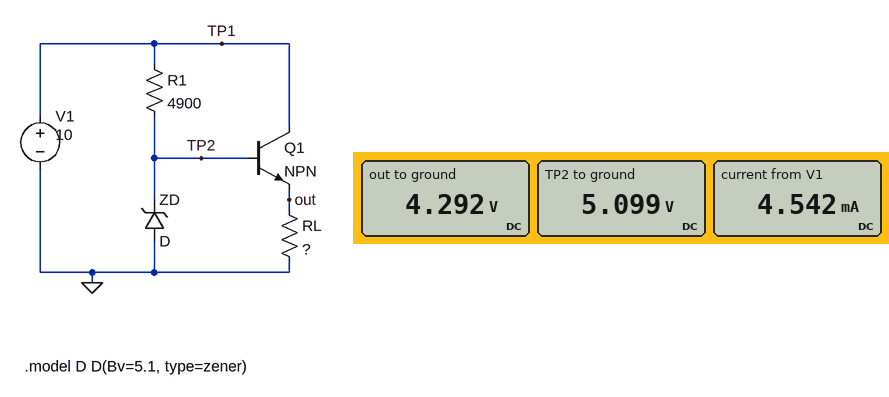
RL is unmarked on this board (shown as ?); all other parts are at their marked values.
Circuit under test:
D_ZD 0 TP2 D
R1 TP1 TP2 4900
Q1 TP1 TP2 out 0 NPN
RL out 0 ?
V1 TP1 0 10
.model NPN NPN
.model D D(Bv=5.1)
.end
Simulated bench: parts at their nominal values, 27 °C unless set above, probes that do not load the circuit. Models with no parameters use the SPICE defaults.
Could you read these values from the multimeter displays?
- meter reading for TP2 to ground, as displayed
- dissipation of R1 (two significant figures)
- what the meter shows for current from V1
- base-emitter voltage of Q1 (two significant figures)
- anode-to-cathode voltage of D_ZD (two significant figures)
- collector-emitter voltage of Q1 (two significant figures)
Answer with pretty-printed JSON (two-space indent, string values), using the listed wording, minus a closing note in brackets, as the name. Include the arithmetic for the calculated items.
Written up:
{
  "meter reading for TP2 to ground, as displayed": "5.099 V",
  "dissipation of R1": "(10 V - 5.099 V)^2 / 4.9 kΩ = 4.9 mW",
  "what the meter shows for current from V1": "4.542 mA",
  "base-emitter voltage of Q1": "5.099 V - 4.292 V = 810 mV",
  "anode-to-cathode voltage of D_ZD": "0 V - 5.099 V = -5.1 V",
  "collector-emitter voltage of Q1": "10 V - 4.292 V = 5.7 V"
}
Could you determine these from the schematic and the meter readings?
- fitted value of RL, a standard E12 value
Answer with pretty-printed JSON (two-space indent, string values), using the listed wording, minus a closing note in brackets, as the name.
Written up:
{
  "fitted value of RL, a standard E12 value": "1.2 kΩ"
}
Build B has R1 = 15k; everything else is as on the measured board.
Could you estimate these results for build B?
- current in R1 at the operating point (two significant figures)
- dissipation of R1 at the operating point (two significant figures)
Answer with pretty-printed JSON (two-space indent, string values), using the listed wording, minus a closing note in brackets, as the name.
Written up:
{
  "current in R1 at the operating point": "330 µA",
  "dissipation of R1 at the operating point": "1.6 mW"
}
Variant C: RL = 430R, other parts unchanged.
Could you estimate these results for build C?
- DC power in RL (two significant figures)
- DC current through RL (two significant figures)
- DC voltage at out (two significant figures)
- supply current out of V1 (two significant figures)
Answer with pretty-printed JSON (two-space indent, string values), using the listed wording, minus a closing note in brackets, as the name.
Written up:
{
  "DC power in RL": "42 mW",
  "DC current through RL": "9.9 mA",
  "DC voltage at out": "4.3 V",
  "supply current out of V1": "11 mA"
}
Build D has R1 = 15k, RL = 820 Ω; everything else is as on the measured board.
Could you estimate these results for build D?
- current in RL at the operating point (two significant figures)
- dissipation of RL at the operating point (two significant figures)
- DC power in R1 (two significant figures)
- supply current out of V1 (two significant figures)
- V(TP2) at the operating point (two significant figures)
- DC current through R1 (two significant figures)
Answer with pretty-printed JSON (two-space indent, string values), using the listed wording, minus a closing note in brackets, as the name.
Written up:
{
  "current in RL at the operating point": "5.2 mA",
  "dissipation of RL at the operating point": "22 mW",
  "DC power in R1": "1.6 mW",
  "supply current out of V1": "5.5 mA",
  "V(TP2) at the operating point": "5.1 V",
  "DC current through R1": "330 µA"
}
